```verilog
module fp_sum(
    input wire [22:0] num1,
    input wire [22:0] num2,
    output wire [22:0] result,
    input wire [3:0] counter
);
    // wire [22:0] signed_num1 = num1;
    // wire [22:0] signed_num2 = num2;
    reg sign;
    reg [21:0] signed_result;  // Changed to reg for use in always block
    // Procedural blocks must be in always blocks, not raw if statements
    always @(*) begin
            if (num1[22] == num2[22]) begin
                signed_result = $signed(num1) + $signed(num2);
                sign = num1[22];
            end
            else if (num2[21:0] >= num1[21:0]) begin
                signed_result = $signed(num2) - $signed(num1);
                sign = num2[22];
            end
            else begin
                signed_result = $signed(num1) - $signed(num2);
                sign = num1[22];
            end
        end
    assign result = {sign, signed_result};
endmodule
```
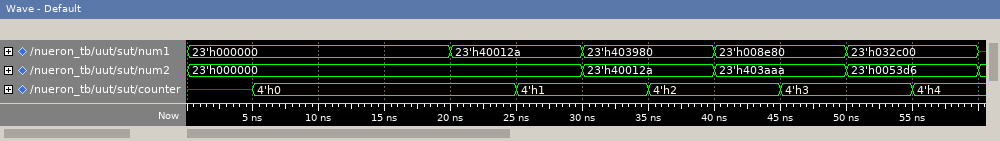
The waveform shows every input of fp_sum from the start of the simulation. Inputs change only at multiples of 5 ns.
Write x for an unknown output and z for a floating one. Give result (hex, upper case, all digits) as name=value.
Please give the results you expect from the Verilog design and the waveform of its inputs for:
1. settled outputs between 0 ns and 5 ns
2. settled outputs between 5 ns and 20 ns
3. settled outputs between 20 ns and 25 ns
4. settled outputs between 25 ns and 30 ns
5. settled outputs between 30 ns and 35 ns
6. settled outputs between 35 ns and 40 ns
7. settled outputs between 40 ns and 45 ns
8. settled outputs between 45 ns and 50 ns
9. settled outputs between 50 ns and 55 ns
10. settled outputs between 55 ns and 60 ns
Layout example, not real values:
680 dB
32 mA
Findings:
result=000000
result=000000
result=40012A
result=40012A
result=403AAA
result=403AAA
result=0053D6
result=0053D6
result=037FD6
result=037FD6
